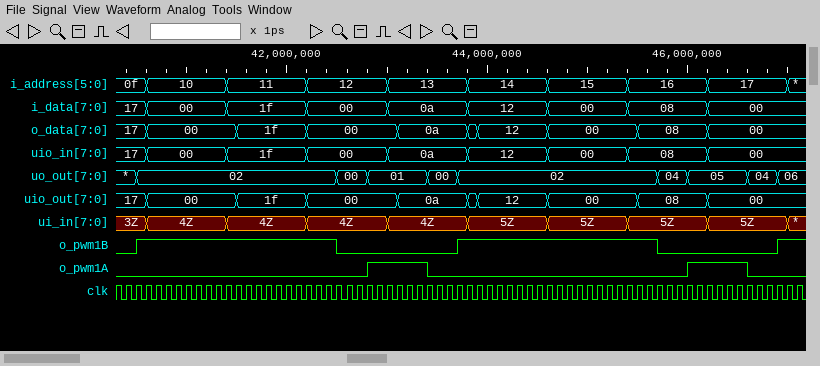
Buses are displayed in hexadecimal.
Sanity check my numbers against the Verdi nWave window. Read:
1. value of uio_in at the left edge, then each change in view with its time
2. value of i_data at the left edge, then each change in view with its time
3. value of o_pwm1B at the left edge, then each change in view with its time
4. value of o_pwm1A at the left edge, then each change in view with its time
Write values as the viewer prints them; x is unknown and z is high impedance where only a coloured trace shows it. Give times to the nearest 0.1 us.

17, 00 at 40.6 us, 1f at 41.4 us, 00 at 42.2 us, 0a at 43 us, 12 at 43.8 us, 00 at 44.6 us, 08 at 45.4 us, 00 at 46.2 us
17, 00 at 40.6 us, 1f at 41.4 us, 00 at 42.2 us, 0a at 43 us, 12 at 43.8 us, 00 at 44.6 us, 08 at 45.4 us, 00 at 46.2 us
0, 1 at 40.5 us, 0 at 42.5 us, 1 at 43.7 us, 0 at 45.7 us, 1 at 46.9 us
0, 1 at 42.8 us, 0 at 43.4 us, 1 at 46 us, 0 at 46.6 us
